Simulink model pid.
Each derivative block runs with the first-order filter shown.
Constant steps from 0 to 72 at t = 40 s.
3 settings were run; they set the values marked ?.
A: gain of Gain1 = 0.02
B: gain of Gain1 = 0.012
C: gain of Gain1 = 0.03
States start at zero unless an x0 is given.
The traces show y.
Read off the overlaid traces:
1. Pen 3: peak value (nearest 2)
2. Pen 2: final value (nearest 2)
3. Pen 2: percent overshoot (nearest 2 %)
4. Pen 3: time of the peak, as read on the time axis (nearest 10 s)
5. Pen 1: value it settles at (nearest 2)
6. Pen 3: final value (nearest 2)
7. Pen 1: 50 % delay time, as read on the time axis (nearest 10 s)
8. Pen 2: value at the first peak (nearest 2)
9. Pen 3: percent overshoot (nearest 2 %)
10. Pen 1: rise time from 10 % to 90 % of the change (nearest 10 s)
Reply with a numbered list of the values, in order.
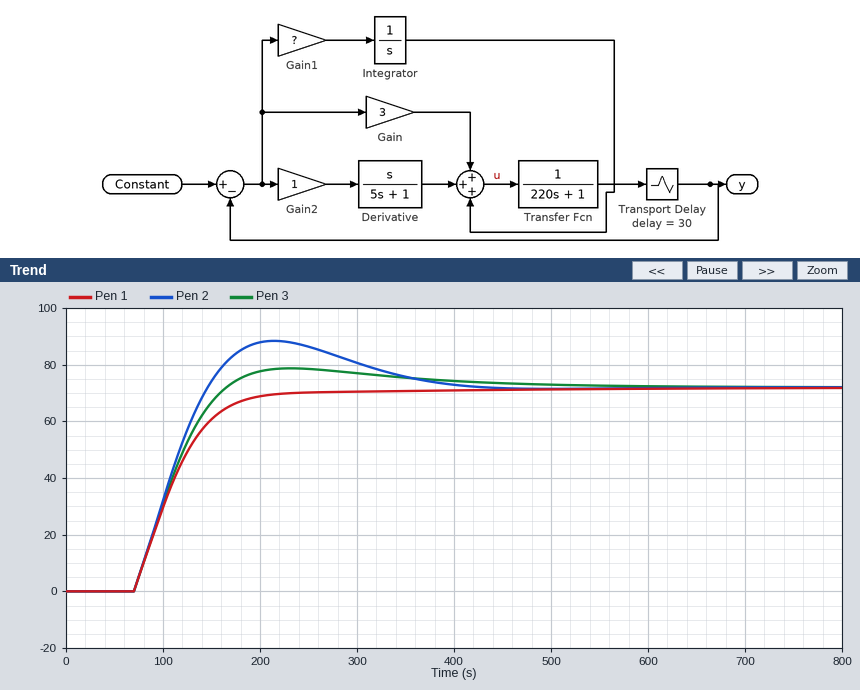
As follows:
1. 78
2. 72
3. 22 %
4. 230 s
5. 72
6. 72
7. 110 s
8. 88
9. 10 %
10. 90 s
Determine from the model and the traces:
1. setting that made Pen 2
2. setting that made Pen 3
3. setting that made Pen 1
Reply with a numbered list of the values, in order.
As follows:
1. C
2. A
3. B
